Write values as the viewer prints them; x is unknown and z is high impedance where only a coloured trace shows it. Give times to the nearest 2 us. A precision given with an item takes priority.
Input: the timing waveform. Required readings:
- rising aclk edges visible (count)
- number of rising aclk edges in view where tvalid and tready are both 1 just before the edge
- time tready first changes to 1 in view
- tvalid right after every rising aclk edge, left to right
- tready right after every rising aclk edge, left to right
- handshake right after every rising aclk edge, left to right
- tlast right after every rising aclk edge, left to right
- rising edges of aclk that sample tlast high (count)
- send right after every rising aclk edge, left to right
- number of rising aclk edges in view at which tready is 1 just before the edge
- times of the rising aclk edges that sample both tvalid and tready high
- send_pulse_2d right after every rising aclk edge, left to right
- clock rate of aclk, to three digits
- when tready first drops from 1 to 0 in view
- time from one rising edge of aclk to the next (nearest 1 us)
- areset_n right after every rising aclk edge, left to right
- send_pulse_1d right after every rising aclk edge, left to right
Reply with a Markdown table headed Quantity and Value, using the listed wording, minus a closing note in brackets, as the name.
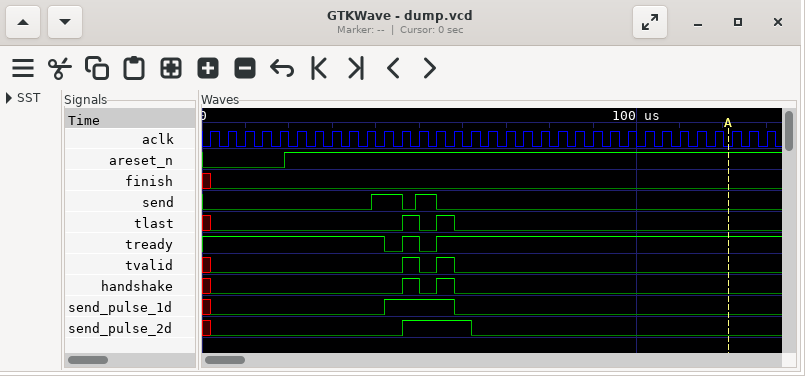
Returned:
| Quantity | Value |
|---|---|
| rising aclk edges visible | 33 |
| number of rising aclk edges in view where tvalid and tready are both 1 just before the edge | 2 |
| time tready first changes to 1 in view | 46 us |
| tvalid right after every rising aclk edge, left to right | 0 0 0 0 0 0 0 0 0 0 0 1 0 1 0 0 0 0 0 0 0 0 0 0 0 0 0 0 0 0 0 0 0 |
| tready right after every rising aclk edge, left to right | 1 1 1 1 1 1 1 1 1 1 0 1 0 1 1 1 1 1 1 1 1 1 1 1 1 1 1 1 1 1 1 1 1 |
| handshake right after every rising aclk edge, left to right | 0 0 0 0 0 0 0 0 0 0 0 1 0 1 0 0 0 0 0 0 0 0 0 0 0 0 0 0 0 0 0 0 0 |
| tlast right after every rising aclk edge, left to right | 0 0 0 0 0 0 0 0 0 0 0 1 0 1 0 0 0 0 0 0 0 0 0 0 0 0 0 0 0 0 0 0 0 |
| rising edges of aclk that sample tlast high | 2 |
| send right after every rising aclk edge, left to right | 0 0 0 0 0 0 0 0 0 0 1 0 1 0 0 0 0 0 0 0 0 0 0 0 0 0 0 0 0 0 0 0 0 |
| number of rising aclk edges in view at which tready is 1 just before the edge | 31 |
| times of the rising aclk edges that sample both tvalid and tready high | 50 us, 58 us |
| send_pulse_2d right after every rising aclk edge, left to right | 0 0 0 0 0 0 0 0 0 0 0 1 1 1 1 0 0 0 0 0 0 0 0 0 0 0 0 0 0 0 0 0 0 |
| clock rate of aclk, to three digits | 250 kHz |
| when tready first drops from 1 to 0 in view | 42 us |
| time from one rising edge of aclk to the next | 4 us |
| areset_n right after every rising aclk edge, left to right | 0 0 0 0 0 1 1 1 1 1 1 1 1 1 1 1 1 1 1 1 1 1 1 1 1 1 1 1 1 1 1 1 1 |
| send_pulse_1d right after every rising aclk edge, left to right | 0 0 0 0 0 0 0 0 0 0 1 1 1 1 0 0 0 0 0 0 0 0 0 0 0 0 0 0 0 0 0 0 0 |
